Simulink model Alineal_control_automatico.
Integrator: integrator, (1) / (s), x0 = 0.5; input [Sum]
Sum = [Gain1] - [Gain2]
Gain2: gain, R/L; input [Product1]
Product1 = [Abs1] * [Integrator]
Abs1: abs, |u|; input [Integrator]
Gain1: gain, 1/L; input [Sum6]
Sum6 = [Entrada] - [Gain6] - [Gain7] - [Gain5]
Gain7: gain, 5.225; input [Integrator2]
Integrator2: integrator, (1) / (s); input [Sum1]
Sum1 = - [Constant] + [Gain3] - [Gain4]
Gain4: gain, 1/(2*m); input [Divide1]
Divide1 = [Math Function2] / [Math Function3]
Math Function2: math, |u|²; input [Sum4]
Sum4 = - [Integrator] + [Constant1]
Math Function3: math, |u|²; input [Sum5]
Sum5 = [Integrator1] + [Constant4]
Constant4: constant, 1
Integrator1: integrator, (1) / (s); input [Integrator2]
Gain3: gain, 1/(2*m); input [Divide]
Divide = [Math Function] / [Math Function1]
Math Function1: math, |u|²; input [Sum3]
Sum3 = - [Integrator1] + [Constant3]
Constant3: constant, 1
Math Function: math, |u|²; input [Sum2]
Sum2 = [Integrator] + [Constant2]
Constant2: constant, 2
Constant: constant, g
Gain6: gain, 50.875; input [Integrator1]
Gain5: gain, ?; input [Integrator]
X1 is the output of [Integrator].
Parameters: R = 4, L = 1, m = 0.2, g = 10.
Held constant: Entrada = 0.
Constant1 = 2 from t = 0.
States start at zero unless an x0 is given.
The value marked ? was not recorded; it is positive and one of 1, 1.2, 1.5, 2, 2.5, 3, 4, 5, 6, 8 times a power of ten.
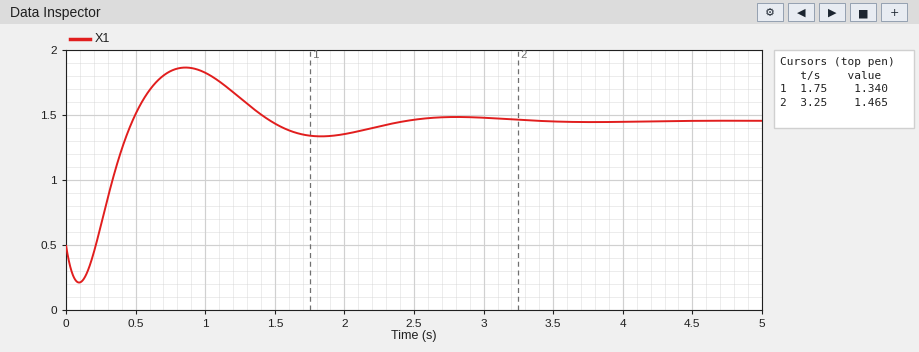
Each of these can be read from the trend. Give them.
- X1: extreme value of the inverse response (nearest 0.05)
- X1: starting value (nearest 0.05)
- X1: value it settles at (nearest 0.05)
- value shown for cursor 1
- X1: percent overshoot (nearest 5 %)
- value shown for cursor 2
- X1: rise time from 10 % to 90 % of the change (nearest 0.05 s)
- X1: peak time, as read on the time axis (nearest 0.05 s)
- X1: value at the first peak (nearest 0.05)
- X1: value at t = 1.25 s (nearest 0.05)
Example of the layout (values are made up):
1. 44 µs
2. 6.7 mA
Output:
1. 0.20
2. 0.50
3. 1.45
4. 1.340
5. 45 %
6. 1.465
7. 0.20 s
8. 0.85 s
9. 1.85
10. 1.65
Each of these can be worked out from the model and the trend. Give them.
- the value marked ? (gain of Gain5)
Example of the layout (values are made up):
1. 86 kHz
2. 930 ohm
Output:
1. 12
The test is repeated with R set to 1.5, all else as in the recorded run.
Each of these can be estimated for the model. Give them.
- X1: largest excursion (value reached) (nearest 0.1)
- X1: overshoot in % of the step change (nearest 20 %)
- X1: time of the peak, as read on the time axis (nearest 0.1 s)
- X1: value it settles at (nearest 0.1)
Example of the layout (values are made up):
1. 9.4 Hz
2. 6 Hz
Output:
1. 1.6
2. 100 %
3. 0.6 s
4. 1.1
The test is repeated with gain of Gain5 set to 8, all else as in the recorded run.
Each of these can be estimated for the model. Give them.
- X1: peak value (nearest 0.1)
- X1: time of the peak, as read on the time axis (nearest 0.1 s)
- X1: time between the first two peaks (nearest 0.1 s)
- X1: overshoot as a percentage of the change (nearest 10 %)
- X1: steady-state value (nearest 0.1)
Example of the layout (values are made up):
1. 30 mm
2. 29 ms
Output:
1. 1.4
2. 0.6 s
3. 1.2 s
4. 100 %
5. 0.9
